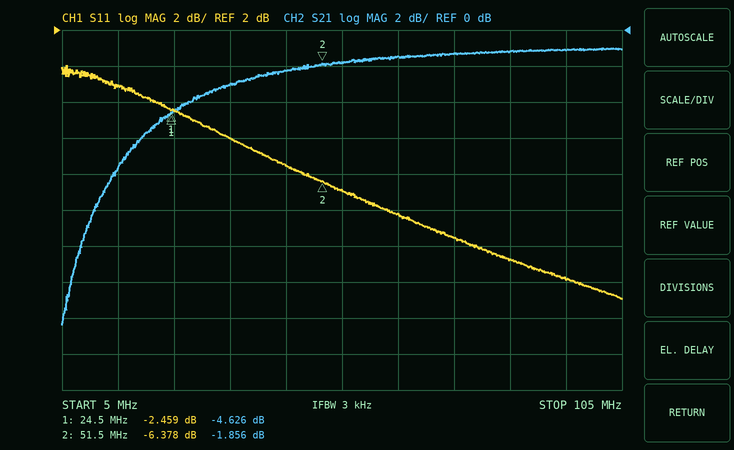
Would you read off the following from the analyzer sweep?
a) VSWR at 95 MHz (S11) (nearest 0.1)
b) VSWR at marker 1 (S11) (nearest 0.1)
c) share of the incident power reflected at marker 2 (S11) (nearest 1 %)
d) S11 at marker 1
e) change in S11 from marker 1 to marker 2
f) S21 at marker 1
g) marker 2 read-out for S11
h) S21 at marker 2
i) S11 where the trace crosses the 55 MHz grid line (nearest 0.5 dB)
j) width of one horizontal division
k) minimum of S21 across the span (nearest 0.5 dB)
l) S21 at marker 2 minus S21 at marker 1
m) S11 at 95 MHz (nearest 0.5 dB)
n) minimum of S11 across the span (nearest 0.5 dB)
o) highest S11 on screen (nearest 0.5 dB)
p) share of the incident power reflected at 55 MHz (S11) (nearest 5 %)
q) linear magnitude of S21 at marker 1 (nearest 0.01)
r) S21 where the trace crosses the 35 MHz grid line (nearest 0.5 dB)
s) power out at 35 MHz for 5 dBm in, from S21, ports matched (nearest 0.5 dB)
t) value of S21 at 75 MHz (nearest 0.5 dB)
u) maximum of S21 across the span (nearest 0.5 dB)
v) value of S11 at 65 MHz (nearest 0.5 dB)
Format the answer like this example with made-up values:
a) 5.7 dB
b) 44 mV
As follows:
a) 1.7
b) 7.1
c) 23 %
d) -2.459 dB
e) -3.919 dB
f) -4.626 dB
g) -6.378 dB
h) -1.856 dB
i) -7.0 dB
j) 10 MHz
k) -16.5 dB
l) 2.770 dB
m) -12.0 dB
n) -13.0 dB
o) 0.0 dB
p) 20 %
q) 0.59
r) -3.0 dB
s) 2.0 dBm
t) -1.5 dB
u) -1.0 dB
v) -8.0 dB
